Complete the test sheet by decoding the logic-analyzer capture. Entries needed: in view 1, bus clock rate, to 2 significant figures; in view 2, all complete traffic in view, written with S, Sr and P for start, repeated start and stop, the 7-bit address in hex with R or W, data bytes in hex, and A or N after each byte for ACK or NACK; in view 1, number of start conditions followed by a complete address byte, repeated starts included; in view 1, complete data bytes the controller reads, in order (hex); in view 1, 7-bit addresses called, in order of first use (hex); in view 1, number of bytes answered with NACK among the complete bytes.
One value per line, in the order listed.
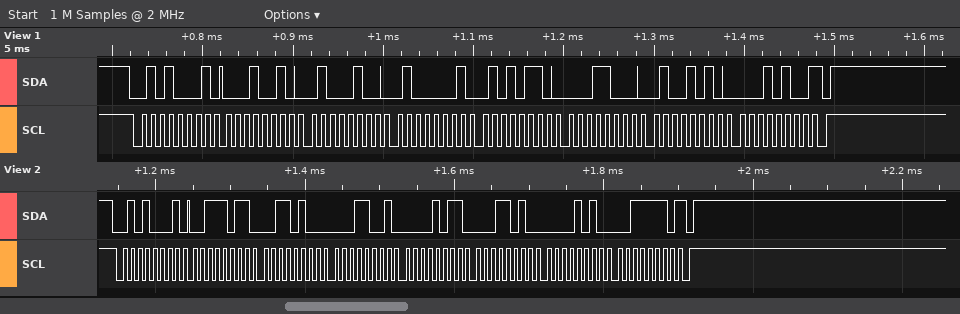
100 kHz
S 28R A 3B A 34 A 19 A 0B A 1A A 0A A 3E N P
1
12 44 41 56 18 4A 14
0x28
1
